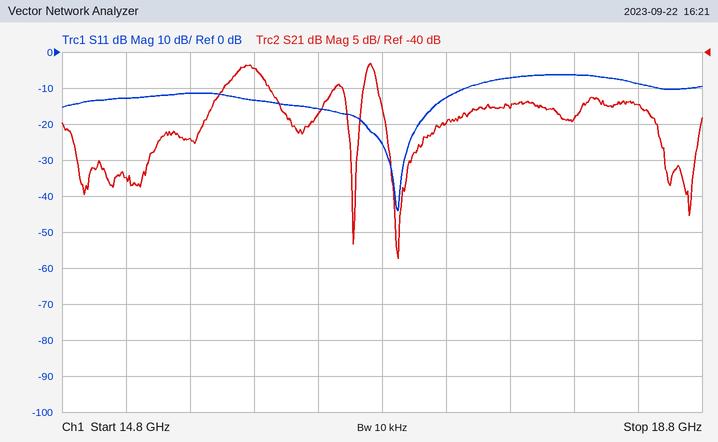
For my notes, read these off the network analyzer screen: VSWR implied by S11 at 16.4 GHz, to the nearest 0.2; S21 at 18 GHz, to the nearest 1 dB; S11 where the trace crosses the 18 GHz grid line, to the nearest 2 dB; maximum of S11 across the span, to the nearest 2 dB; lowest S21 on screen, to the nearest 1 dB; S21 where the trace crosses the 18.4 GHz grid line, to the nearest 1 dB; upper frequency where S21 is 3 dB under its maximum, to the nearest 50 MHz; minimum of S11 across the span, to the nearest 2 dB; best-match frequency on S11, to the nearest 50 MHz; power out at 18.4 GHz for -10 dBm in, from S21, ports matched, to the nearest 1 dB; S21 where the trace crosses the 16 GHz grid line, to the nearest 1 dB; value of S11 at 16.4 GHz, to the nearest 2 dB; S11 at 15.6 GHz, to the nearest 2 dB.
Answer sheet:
1.4
-49 dB
-6 dB
-6 dB
-69 dB
-47 dB
16.75 GHz
-44 dB
16.90 GHz
-57 dBm
-42 dB
-16 dB
-12 dB
